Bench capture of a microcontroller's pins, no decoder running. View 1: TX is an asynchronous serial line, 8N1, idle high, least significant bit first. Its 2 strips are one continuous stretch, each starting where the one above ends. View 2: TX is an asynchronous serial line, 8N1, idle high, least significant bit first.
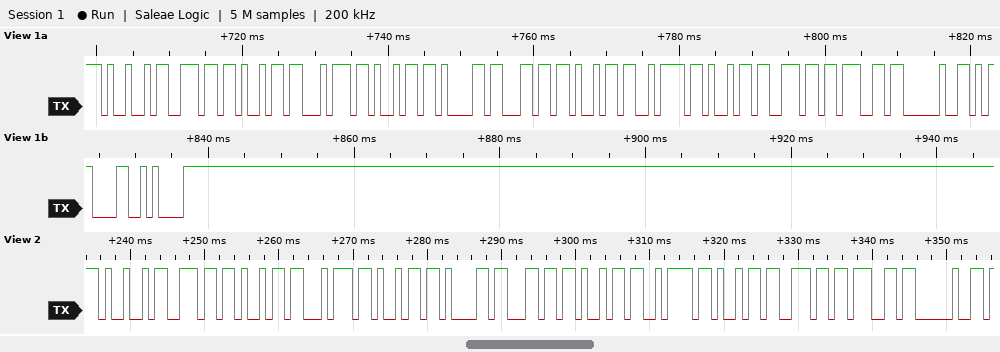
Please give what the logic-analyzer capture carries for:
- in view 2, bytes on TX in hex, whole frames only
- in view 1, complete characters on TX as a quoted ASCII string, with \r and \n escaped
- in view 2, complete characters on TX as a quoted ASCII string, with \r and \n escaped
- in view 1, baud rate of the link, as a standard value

49 6E 69 74 69 61 6C 69 7A 69 6E 67 20
"Initializing \r\n"
"Initializing "
1200 baud
